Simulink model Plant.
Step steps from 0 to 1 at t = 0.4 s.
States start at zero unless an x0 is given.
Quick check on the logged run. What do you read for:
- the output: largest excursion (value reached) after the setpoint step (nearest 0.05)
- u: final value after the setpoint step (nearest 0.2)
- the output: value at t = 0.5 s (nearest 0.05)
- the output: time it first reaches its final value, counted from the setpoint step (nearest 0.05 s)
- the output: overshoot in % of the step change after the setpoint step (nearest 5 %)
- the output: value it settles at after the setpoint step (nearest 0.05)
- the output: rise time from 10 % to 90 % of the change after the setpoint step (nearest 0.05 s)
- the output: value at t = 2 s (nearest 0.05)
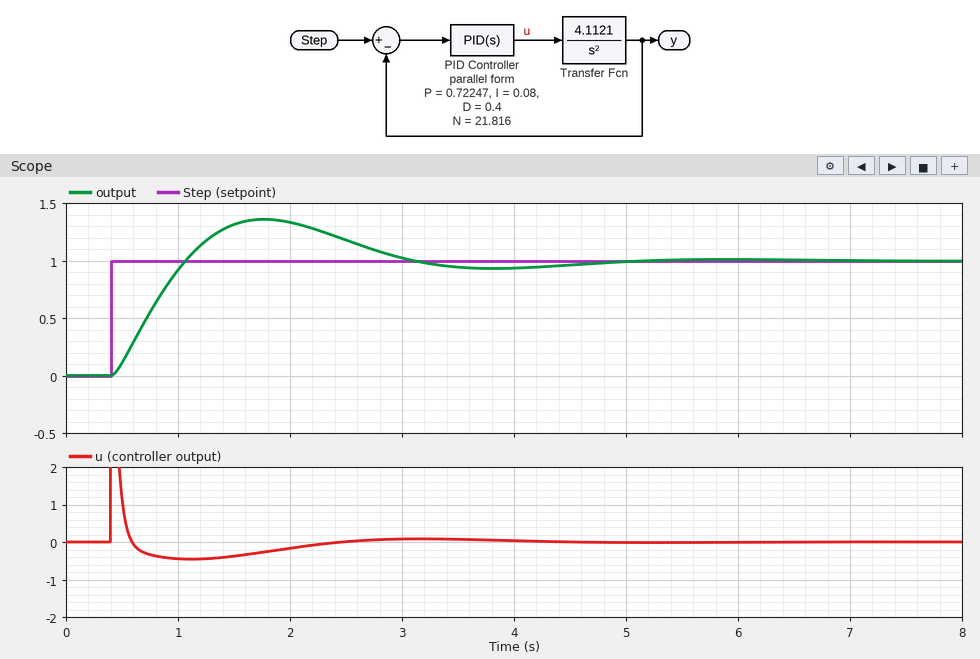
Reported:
1.35
0.0
0.10
0.65 s
35 %
1.00
0.50 s
1.35
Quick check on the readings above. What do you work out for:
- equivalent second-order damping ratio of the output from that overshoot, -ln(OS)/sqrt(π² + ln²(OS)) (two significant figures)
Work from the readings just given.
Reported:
0.32
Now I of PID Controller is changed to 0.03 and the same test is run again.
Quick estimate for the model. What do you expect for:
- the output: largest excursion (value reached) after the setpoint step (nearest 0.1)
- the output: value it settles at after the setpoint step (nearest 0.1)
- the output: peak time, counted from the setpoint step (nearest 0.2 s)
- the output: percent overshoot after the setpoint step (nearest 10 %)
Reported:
1.3
1.0
1.4 s
30 %
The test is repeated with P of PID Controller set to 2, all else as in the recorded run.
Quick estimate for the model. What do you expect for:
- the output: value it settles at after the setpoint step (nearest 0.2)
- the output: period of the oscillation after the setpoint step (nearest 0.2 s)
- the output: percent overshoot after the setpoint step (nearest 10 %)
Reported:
1.0
2.2 s
50 %
